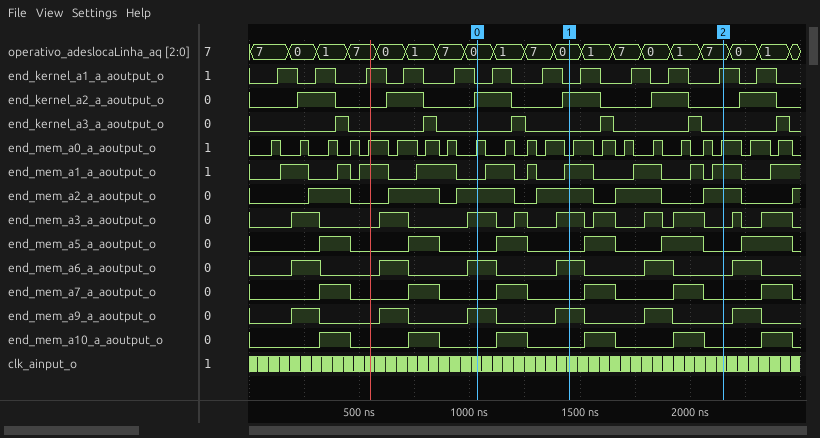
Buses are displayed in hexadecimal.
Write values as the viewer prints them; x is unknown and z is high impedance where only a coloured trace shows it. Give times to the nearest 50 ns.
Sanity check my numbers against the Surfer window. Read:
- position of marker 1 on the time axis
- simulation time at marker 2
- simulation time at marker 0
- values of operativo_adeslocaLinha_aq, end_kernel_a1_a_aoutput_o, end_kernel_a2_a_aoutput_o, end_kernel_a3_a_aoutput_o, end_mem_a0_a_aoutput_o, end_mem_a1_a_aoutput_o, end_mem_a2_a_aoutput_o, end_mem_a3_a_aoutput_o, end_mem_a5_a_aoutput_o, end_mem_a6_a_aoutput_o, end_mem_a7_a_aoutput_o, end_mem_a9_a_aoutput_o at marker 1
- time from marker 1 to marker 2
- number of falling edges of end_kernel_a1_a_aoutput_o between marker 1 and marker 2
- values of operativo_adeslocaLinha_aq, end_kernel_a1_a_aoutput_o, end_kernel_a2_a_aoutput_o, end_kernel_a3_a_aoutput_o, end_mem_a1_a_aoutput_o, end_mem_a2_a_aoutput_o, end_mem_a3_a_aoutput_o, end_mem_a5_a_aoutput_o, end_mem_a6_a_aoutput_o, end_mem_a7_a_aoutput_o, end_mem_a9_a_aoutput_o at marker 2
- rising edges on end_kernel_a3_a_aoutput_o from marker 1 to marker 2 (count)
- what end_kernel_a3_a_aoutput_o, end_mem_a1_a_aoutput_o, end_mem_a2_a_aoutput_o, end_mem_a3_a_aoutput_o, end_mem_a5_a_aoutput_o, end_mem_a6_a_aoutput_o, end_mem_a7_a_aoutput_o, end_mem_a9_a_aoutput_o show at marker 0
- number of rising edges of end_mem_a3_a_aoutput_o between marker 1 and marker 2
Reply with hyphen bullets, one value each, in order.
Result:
- 1450 ns
- 2150 ns
- 1050 ns
- operativo_adeslocaLinha_aq=0, end_kernel_a1_a_aoutput_o=0, end_kernel_a2_a_aoutput_o=1, end_kernel_a3_a_aoutput_o=0, end_mem_a0_a_aoutput_o=0, end_mem_a1_a_aoutput_o=1, end_mem_a2_a_aoutput_o=1, end_mem_a3_a_aoutput_o=1, end_mem_a5_a_aoutput_o=0, end_mem_a6_a_aoutput_o=1, end_mem_a7_a_aoutput_o=0, end_mem_a9_a_aoutput_o=1
- 700 ns
- 3
- operativo_adeslocaLinha_aq=7, end_kernel_a1_a_aoutput_o=1, end_kernel_a2_a_aoutput_o=0, end_kernel_a3_a_aoutput_o=0, end_mem_a1_a_aoutput_o=1, end_mem_a2_a_aoutput_o=1, end_mem_a3_a_aoutput_o=0, end_mem_a5_a_aoutput_o=0, end_mem_a6_a_aoutput_o=0, end_mem_a7_a_aoutput_o=0, end_mem_a9_a_aoutput_o=0
- 2
- end_kernel_a3_a_aoutput_o=0, end_mem_a1_a_aoutput_o=0, end_mem_a2_a_aoutput_o=1, end_mem_a3_a_aoutput_o=1, end_mem_a5_a_aoutput_o=0, end_mem_a6_a_aoutput_o=1, end_mem_a7_a_aoutput_o=0, end_mem_a9_a_aoutput_o=1
- 3
